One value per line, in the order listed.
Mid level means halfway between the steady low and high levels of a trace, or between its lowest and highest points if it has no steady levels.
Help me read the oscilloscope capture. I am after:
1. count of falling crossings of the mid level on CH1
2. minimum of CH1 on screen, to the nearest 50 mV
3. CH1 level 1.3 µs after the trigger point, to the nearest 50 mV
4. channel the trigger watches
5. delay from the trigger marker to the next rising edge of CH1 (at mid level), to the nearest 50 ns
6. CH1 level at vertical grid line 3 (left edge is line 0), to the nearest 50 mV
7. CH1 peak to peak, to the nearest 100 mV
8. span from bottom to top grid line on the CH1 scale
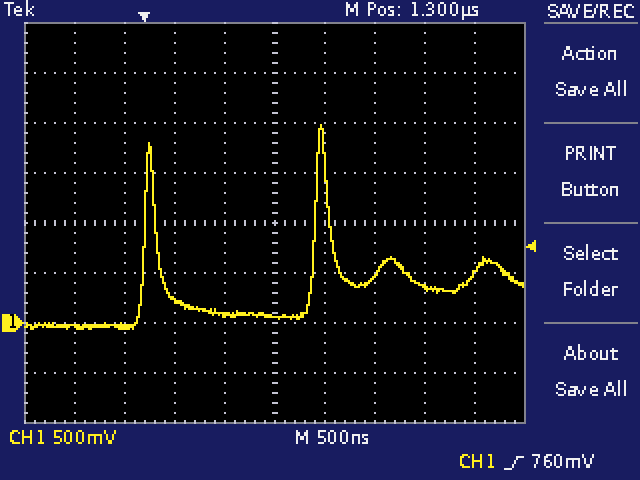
2
-50 mV
50 mV
CH1
1.70 µs
250 mV
2.00 V
4 V
